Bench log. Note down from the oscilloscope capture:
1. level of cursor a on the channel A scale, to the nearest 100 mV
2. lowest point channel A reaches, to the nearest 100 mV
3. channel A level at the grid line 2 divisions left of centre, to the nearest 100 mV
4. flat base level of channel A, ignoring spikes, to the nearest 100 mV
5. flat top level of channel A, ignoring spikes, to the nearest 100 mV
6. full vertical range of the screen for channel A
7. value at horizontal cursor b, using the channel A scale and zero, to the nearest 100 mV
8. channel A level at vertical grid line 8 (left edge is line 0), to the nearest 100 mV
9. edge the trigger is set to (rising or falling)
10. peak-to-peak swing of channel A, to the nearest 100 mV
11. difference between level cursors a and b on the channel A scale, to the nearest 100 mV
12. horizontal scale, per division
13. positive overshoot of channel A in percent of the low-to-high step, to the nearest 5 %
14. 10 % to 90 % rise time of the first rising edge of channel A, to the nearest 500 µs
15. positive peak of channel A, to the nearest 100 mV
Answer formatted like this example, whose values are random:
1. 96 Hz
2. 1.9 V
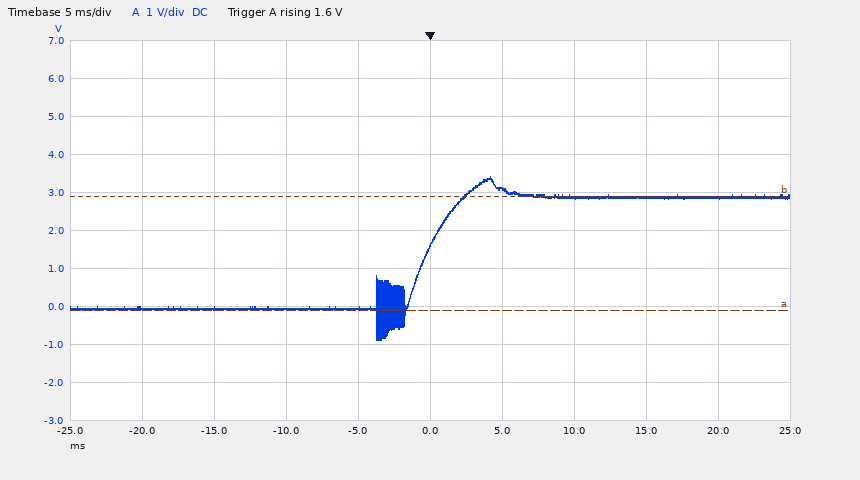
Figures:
1. -100 mV
2. -900 mV
3. -100 mV
4. -100 mV
5. 2.9 V
6. 10 V
7. 2.9 V
8. 2.9 V
9. rising
10. 4.3 V
11. 3.0 V
12. 5 ms
13. 20 %
14. 3.0 ms
15. 3.4 V
